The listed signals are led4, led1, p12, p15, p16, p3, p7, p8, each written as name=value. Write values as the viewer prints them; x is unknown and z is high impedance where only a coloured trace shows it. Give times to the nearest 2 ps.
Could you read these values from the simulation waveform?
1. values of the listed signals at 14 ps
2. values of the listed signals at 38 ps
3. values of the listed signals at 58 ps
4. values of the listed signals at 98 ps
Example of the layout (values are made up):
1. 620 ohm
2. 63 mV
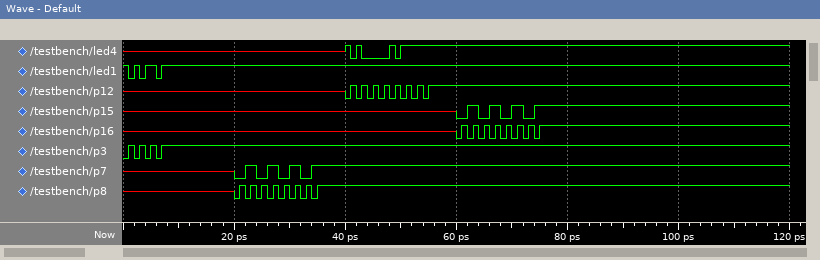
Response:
1. led4=x, led1=1, p12=x, p15=x, p16=x, p3=1, p7=x, p8=x
2. led4=x, led1=1, p12=x, p15=x, p16=x, p3=1, p7=1, p8=1
3. led4=1, led1=1, p12=1, p15=x, p16=x, p3=1, p7=1, p8=1
4. led4=1, led1=1, p12=1, p15=1, p16=1, p3=1, p7=1, p8=1
